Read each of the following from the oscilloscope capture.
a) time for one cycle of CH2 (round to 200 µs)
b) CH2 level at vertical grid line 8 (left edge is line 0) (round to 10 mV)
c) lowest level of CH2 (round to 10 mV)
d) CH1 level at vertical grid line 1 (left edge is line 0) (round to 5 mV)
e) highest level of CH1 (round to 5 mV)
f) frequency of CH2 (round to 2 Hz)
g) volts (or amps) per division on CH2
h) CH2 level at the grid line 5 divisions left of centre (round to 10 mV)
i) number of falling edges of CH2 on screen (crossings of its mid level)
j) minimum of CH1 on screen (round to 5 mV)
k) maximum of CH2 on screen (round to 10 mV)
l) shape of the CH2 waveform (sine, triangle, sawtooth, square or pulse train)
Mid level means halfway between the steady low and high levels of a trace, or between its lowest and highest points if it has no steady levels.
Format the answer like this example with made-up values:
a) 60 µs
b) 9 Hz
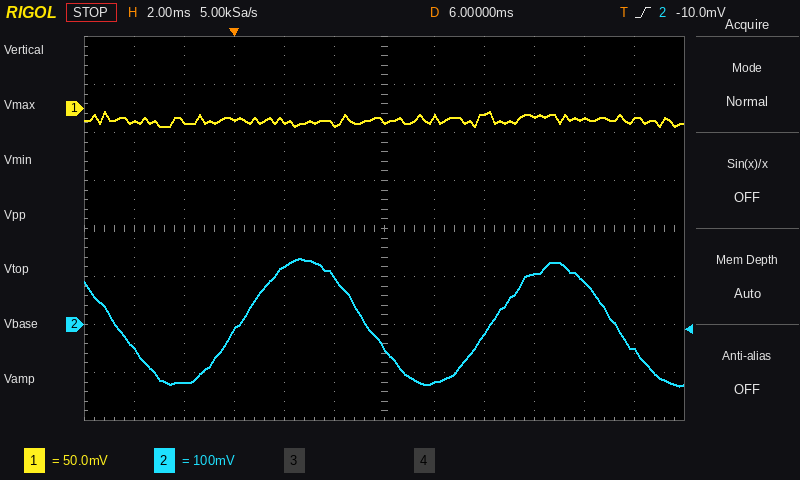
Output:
a) 10.0 ms
b) -20 mV
c) -130 mV
d) -15 mV
e) -5 mV
f) 100 Hz
g) 100 mV
h) -50 mV
i) 3
j) -20 mV
k) 140 mV
l) sine
